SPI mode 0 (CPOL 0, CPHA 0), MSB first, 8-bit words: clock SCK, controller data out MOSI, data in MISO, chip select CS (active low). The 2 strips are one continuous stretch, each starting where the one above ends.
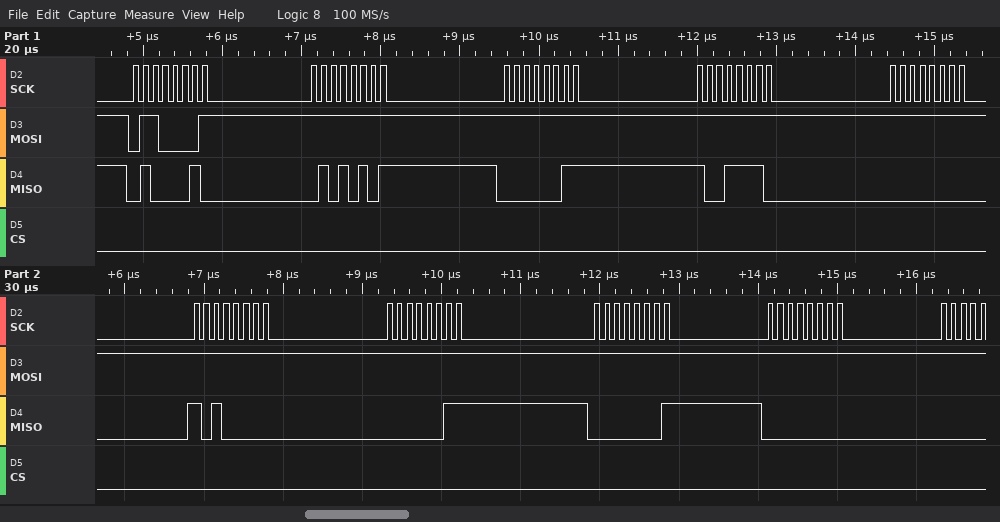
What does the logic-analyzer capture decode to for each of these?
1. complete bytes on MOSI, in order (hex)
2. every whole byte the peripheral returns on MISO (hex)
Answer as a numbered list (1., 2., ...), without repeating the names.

1. 61 FF FF FF FF FF FF FF FF
2. 42 55 03 9E 00 A0 03 01 00
